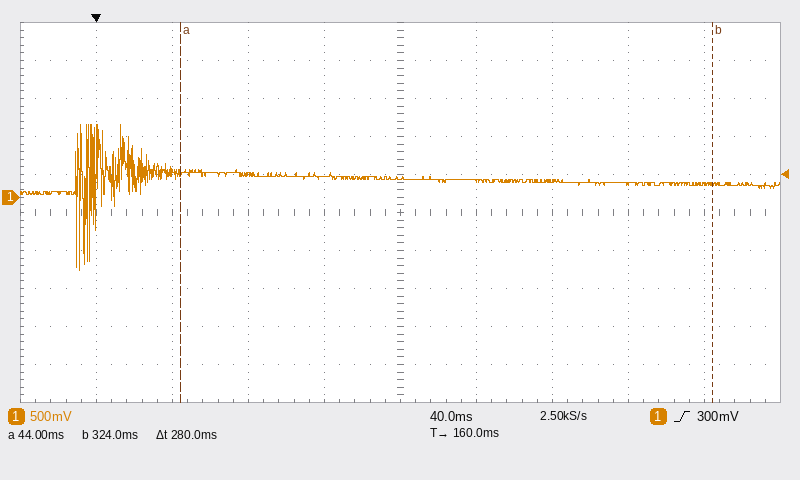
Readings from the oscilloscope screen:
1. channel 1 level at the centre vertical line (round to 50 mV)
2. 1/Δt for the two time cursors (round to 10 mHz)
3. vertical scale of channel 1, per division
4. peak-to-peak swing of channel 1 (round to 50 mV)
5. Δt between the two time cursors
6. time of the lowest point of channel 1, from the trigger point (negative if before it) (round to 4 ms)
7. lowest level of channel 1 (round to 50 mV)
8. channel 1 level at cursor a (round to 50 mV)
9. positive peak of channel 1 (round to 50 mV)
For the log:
250 mV
3.57 Hz
500 mV
1.90 V
280 ms
-8 ms
-950 mV
300 mV
950 mV
